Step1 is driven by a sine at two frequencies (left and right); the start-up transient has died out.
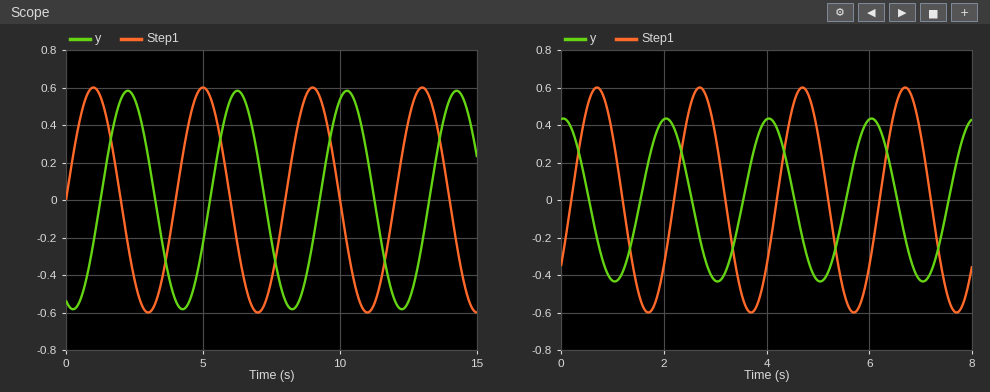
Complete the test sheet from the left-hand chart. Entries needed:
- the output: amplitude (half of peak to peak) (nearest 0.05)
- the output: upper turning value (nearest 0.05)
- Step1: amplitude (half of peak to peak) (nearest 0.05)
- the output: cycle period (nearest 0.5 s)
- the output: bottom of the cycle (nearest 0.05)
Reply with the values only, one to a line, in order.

0.60
0.60
0.60
4.0 s
-0.60
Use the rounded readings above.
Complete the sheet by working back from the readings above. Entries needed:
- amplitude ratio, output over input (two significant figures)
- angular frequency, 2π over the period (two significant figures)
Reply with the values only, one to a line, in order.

1.0
1.6 rad/s
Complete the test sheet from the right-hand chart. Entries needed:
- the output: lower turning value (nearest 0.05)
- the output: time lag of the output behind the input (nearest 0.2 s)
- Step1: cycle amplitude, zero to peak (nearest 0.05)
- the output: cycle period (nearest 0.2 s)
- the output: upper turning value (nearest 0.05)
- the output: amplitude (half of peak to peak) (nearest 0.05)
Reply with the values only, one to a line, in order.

-0.45
1.4 s
0.60
2.0 s
0.45
0.45
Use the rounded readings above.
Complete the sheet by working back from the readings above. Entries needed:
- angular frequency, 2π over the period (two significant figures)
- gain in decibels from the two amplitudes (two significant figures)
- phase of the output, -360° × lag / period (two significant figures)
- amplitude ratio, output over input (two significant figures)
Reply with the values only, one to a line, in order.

3.1 rad/s
-2.5 dB
-250°
0.75
